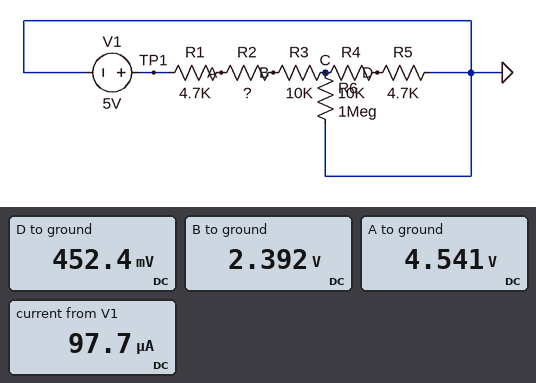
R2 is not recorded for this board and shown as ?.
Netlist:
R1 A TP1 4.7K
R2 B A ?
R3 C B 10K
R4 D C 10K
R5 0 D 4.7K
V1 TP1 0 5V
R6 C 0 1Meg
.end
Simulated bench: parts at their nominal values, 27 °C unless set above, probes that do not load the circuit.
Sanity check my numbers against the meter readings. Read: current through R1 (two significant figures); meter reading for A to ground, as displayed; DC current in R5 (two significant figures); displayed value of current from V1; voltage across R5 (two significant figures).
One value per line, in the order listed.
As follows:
98 µA
4.541 V
96 µA
97.7 µA
450 mV
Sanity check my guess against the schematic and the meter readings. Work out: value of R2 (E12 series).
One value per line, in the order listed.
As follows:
22 kΩ
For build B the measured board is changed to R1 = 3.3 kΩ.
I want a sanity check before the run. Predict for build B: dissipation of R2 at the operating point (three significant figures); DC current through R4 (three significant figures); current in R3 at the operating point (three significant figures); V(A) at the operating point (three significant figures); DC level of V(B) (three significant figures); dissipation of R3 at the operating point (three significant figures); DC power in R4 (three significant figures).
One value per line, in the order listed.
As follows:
222 µW
99.0 µA
100 µA
4.67 V
2.46 V
101 µW
98.0 µW
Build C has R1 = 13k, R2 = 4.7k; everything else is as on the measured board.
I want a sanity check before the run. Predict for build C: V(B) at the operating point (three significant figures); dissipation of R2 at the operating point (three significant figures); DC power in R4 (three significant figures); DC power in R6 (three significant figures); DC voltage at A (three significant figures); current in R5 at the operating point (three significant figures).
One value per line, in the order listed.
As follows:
2.90 V
66.0 µW
136 µW
2.95 µW
3.46 V
117 µA
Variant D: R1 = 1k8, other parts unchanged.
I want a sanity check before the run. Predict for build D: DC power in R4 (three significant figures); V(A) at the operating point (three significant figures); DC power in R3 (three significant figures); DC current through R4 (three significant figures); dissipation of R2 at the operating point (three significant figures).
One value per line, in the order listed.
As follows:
104 µW
4.81 V
107 µW
102 µA
236 µW
